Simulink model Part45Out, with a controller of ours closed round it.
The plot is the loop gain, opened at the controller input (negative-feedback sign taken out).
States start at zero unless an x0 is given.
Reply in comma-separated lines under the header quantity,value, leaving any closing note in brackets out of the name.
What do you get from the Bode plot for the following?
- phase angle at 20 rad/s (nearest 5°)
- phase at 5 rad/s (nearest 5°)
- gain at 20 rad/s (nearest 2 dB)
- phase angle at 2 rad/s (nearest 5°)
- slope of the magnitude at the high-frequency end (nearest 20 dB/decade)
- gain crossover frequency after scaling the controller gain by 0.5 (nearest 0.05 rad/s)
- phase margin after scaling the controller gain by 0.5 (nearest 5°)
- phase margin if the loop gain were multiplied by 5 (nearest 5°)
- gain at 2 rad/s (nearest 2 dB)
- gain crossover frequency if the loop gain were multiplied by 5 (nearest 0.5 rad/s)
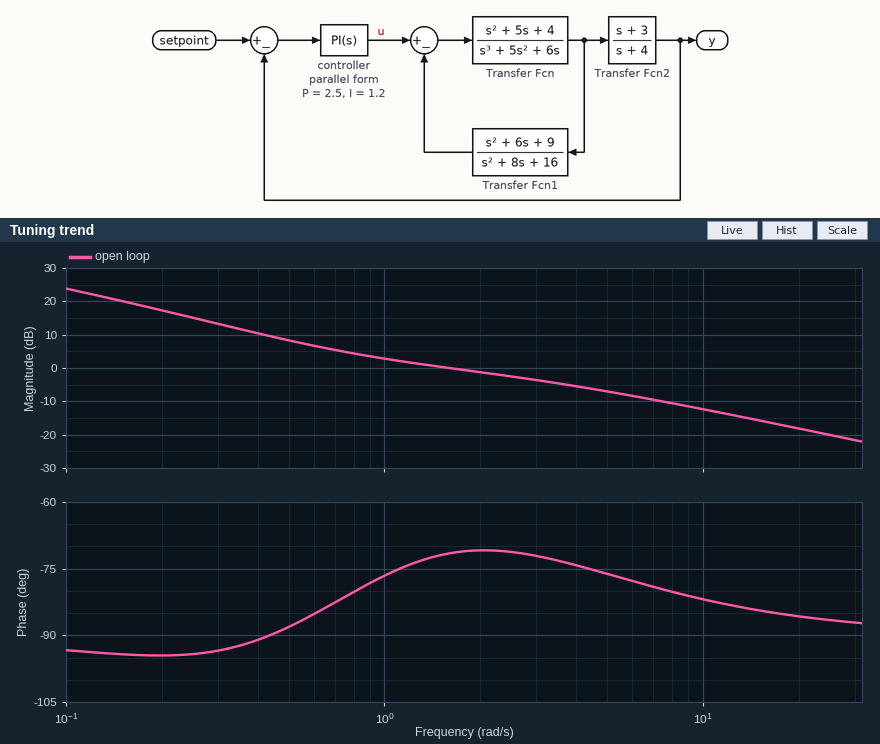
quantity,value
phase angle at 20 rad/s,-85°
phase at 5 rad/s,-75°
gain at 20 rad/s,-18 dB
phase angle at 2 rad/s,-70°
slope of the magnitude at the high-frequency end,-20 dB/decade
gain crossover frequency after scaling the controller gain by 0.5,0.65 rad/s
phase margin after scaling the controller gain by 0.5,95°
phase margin if the loop gain were multiplied by 5,95°
gain at 2 rad/s,-2 dB
gain crossover frequency if the loop gain were multiplied by 5,12.0 rad/s
